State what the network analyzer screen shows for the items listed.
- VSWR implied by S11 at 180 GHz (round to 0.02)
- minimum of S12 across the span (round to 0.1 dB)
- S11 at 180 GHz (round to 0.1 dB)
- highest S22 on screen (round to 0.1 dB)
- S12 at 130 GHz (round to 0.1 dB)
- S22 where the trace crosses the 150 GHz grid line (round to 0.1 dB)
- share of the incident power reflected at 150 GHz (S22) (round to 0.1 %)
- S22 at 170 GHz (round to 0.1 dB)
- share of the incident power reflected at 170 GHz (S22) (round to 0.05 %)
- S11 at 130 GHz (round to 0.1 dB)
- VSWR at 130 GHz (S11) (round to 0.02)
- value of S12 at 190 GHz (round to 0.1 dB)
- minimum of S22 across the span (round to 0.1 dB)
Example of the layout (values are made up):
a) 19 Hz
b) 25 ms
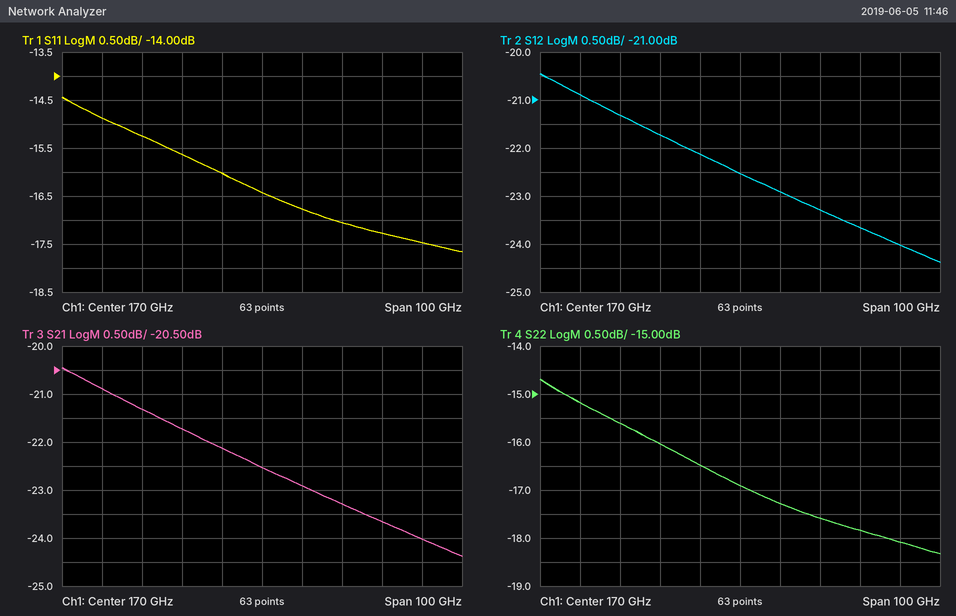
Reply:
a) 1.34
b) -24.4 dB
c) -16.8 dB
d) -14.7 dB
e) -20.9 dB
f) -16.0 dB
g) 2.5 %
h) -16.9 dB
i) 2.05 %
j) -14.9 dB
k) 1.44
l) -23.3 dB
m) -18.3 dB
